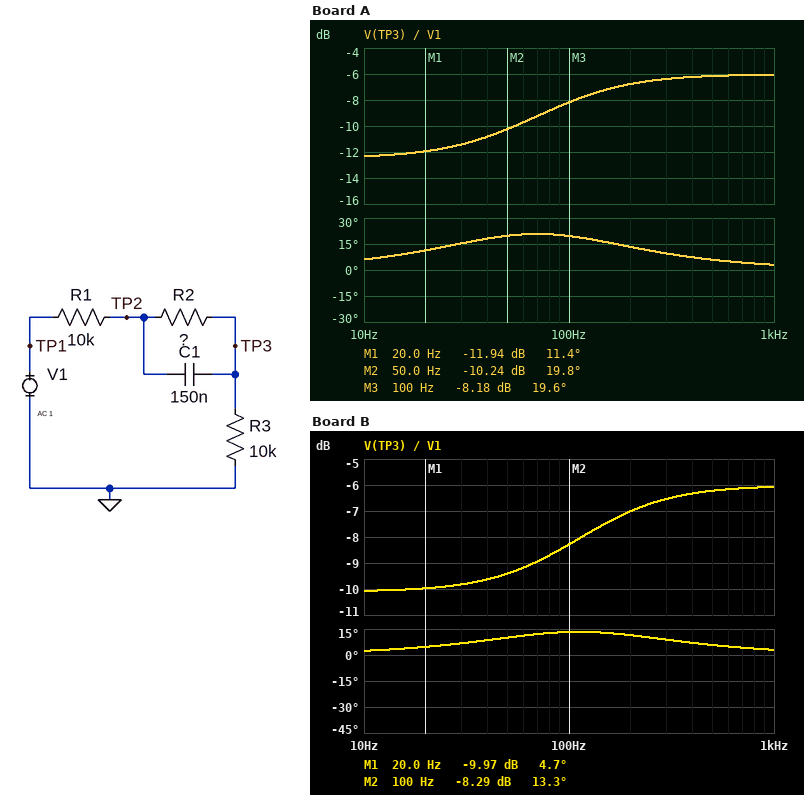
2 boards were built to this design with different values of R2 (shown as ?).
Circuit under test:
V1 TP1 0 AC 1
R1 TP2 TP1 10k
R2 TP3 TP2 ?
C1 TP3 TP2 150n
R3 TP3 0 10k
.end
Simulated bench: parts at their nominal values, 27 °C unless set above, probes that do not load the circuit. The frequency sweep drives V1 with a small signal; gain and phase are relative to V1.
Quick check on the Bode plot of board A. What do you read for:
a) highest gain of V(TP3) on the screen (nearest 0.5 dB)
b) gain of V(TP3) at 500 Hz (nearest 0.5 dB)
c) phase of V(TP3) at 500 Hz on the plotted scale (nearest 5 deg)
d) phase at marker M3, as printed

-6.0 dB
-6.0 dB
5 deg
19.6 deg
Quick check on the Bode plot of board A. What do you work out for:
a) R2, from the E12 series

22 kΩ
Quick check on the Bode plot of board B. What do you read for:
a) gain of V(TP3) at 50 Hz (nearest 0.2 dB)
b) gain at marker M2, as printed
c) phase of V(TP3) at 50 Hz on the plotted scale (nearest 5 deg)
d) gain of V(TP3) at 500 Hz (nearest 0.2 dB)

-9.4 dB
-8.29 dB
10 deg
-6.2 dB
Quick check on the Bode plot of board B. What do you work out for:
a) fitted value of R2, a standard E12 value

12 kΩ
